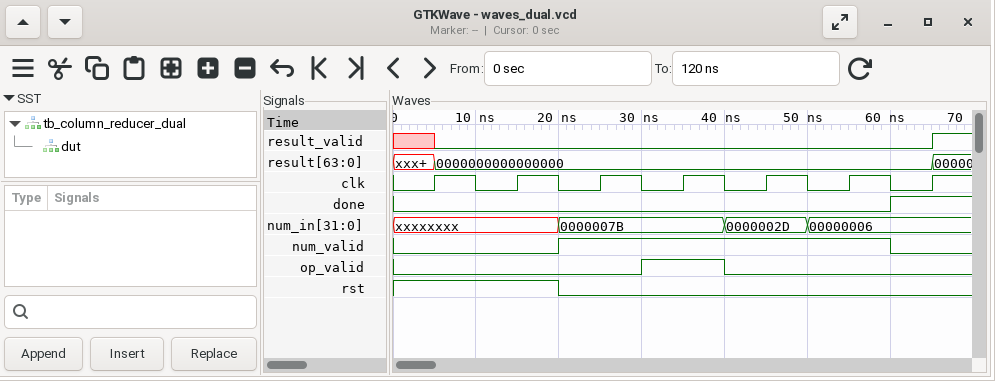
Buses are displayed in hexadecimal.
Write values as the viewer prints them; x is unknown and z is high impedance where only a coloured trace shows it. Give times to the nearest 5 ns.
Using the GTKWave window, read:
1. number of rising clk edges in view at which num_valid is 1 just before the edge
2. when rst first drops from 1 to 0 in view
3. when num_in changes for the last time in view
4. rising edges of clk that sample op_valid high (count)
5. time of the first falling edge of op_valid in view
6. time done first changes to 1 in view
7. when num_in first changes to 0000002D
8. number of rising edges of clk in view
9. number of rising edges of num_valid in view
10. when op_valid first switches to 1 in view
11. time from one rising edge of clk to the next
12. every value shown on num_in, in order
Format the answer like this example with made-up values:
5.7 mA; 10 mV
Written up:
4; 20 ns; 50 ns; 1; 40 ns; 60 ns; 40 ns; 7; 1; 30 ns; 10 ns; xxxxxxxx, 0000007B, 0000002D, 00000006
